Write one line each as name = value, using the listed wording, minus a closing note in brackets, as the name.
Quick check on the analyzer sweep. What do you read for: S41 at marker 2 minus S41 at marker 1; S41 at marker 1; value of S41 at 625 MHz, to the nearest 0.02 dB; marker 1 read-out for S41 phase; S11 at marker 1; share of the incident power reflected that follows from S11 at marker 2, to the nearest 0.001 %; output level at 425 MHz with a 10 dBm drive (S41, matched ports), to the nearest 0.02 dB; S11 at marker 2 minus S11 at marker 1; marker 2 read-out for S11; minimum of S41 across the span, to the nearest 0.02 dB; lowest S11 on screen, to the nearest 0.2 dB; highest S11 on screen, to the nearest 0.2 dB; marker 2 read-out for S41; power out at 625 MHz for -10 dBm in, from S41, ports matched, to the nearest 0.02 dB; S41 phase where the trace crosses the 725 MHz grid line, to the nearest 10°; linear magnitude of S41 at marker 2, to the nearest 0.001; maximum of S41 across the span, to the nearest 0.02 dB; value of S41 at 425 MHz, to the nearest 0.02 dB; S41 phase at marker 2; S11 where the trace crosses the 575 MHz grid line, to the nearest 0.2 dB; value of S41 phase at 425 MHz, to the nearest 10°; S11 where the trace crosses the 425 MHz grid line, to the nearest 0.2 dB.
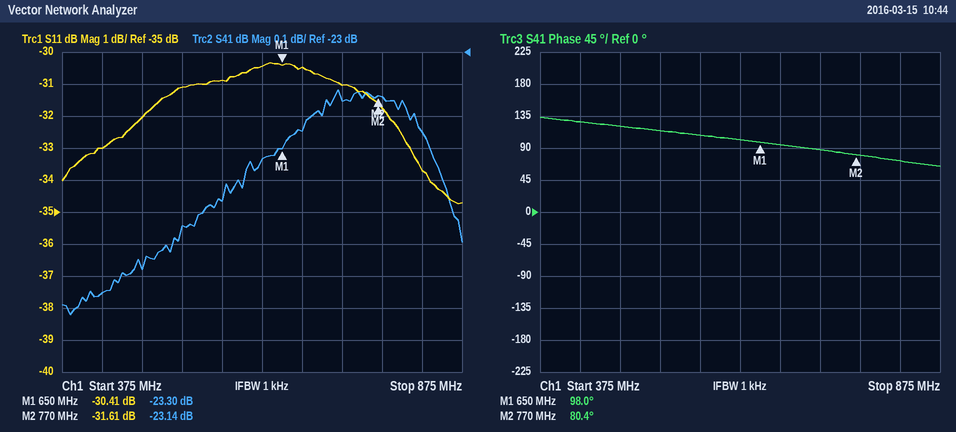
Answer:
S41 at marker 2 minus S41 at marker 1 = 0.16 dB
S41 at marker 1 = -23.30 dB
value of S41 at 625 MHz, to the nearest 0.02 dB = -23.34 dB
marker 1 read-out for S41 phase = 98.0°
S11 at marker 1 = -30.41 dB
share of the incident power reflected that follows from S11 at marker 2, to the nearest 0.001 % = 0.069 %
output level at 425 MHz with a 10 dBm drive (S41, matched ports), to the nearest 0.02 dB = -13.76 dBm
S11 at marker 2 minus S11 at marker 1 = -1.20 dB
marker 2 read-out for S11 = -31.61 dB
minimum of S41 across the span, to the nearest 0.02 dB = -23.82 dB
lowest S11 on screen, to the nearest 0.2 dB = -34.8 dB
highest S11 on screen, to the nearest 0.2 dB = -30.4 dB
marker 2 read-out for S41 = -23.14 dB
power out at 625 MHz for -10 dBm in, from S41, ports matched, to the nearest 0.02 dB = -33.34 dBm
S41 phase where the trace crosses the 725 MHz grid line, to the nearest 10° = 90°
linear magnitude of S41 at marker 2, to the nearest 0.001 = 0.070
maximum of S41 across the span, to the nearest 0.02 dB = -23.12 dB
value of S41 at 425 MHz, to the nearest 0.02 dB = -23.76 dB
S41 phase at marker 2 = 80.4°
S11 where the trace crosses the 575 MHz grid line, to the nearest 0.2 dB = -30.8 dB
value of S41 phase at 425 MHz, to the nearest 10° = 130°
S11 where the trace crosses the 425 MHz grid line, to the nearest 0.2 dB = -33.0 dB
